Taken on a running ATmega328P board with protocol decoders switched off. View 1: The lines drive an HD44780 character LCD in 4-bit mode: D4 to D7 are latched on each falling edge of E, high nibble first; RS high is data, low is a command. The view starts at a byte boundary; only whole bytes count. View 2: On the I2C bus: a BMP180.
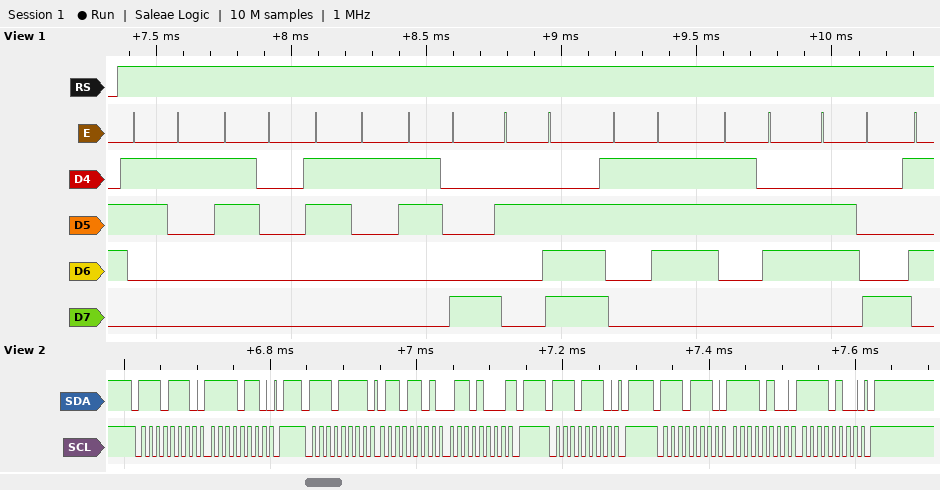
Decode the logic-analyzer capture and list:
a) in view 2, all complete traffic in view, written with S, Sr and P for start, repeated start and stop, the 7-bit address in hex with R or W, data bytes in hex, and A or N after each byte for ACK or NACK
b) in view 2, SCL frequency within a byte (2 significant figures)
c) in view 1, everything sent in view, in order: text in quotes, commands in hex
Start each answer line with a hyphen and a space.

- S 77W A F6 A P S 77R A 6D A 68 N P S 77W A P S 77W A F4 A F4 A P
- 100 kHz
- "1018.76h"
